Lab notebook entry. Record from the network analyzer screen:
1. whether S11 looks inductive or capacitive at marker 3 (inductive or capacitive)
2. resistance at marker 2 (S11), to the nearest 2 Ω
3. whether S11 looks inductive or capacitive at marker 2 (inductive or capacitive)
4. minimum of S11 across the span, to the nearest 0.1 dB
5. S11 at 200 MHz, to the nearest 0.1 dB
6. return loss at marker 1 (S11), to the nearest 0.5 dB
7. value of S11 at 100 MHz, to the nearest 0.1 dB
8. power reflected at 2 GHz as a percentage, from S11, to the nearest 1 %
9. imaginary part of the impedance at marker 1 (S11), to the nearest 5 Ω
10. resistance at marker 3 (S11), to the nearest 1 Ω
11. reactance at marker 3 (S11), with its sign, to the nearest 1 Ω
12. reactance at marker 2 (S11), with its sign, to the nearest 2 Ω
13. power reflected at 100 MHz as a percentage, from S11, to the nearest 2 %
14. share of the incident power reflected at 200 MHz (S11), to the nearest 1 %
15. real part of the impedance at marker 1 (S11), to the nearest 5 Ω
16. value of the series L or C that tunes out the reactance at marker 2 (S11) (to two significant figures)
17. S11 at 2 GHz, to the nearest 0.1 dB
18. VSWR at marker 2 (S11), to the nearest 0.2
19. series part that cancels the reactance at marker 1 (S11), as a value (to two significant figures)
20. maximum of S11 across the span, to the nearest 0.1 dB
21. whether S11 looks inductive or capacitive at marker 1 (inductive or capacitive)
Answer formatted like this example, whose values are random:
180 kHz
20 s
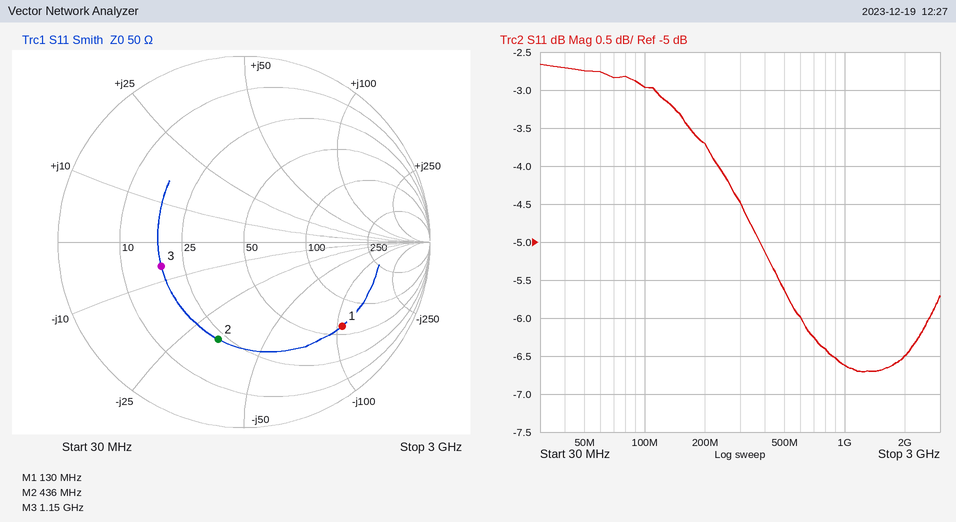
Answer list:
capacitive
22 Ω
capacitive
-6.7 dB
-3.7 dB
3.0 dB
-3.0 dB
22 %
-105 Ω
19 Ω
-6 Ω
-34 Ω
50 %
43 %
60 Ω
12 nH
-6.5 dB
3.4
130 nH
-2.7 dB
capacitive
